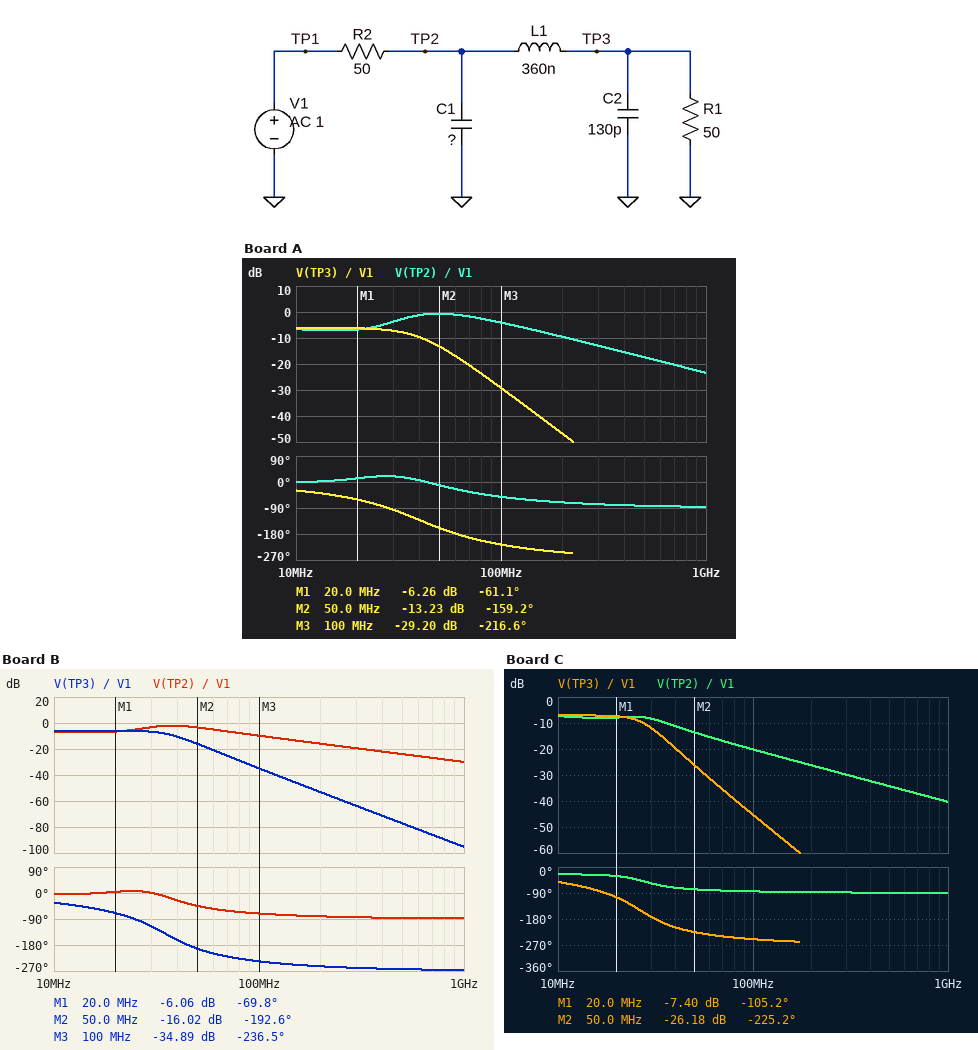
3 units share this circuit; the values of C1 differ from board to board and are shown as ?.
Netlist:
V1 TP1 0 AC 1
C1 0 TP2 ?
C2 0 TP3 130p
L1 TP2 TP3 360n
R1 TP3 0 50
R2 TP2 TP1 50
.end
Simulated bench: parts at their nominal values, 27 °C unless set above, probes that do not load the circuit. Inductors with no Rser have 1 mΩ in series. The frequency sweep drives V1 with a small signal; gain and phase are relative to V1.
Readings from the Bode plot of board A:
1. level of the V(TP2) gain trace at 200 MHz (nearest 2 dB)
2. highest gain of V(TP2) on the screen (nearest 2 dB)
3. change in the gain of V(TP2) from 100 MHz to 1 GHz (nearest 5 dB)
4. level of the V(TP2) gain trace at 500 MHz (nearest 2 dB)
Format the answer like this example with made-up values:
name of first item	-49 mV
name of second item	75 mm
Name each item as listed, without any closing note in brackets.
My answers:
level of the V(TP2) gain trace at 200 MHz	-10 dB
highest gain of V(TP2) on the screen	0 dB
change in the gain of V(TP2) from 100 MHz to 1 GHz	-20 dB
level of the V(TP2) gain trace at 500 MHz	-18 dB
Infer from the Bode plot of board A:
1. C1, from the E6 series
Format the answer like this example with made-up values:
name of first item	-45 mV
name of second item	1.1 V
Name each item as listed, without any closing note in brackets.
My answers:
C1, from the E6 series	47 pF
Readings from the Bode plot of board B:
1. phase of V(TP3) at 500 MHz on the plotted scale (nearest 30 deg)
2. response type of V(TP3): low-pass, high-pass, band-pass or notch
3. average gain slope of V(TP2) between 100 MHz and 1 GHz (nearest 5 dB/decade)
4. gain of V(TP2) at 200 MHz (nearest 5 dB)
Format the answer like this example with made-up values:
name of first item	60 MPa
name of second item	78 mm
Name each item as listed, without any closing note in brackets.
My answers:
phase of V(TP3) at 500 MHz on the plotted scale	-270 deg
response type of V(TP3): low-pass, high-pass, band-pass or notch	low-pass
average gain slope of V(TP2) between 100 MHz and 1 GHz	-20 dB/decade
gain of V(TP2) at 200 MHz	-15 dB
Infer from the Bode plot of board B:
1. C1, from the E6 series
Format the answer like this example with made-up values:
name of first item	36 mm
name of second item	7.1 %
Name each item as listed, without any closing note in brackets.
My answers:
C1, from the E6 series	100 pF
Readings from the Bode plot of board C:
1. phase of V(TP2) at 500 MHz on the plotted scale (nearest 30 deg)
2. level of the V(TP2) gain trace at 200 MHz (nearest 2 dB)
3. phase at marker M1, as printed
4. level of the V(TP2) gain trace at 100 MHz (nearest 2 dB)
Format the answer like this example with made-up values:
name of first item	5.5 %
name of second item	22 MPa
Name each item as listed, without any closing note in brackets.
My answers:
phase of V(TP2) at 500 MHz on the plotted scale	-90 deg
level of the V(TP2) gain trace at 200 MHz	-26 dB
phase at marker M1, as printed	-105.2 deg
level of the V(TP2) gain trace at 100 MHz	-20 dB
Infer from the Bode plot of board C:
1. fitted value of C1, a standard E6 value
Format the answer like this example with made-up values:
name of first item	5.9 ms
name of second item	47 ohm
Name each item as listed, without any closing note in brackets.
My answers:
fitted value of C1, a standard E6 value	330 pF
